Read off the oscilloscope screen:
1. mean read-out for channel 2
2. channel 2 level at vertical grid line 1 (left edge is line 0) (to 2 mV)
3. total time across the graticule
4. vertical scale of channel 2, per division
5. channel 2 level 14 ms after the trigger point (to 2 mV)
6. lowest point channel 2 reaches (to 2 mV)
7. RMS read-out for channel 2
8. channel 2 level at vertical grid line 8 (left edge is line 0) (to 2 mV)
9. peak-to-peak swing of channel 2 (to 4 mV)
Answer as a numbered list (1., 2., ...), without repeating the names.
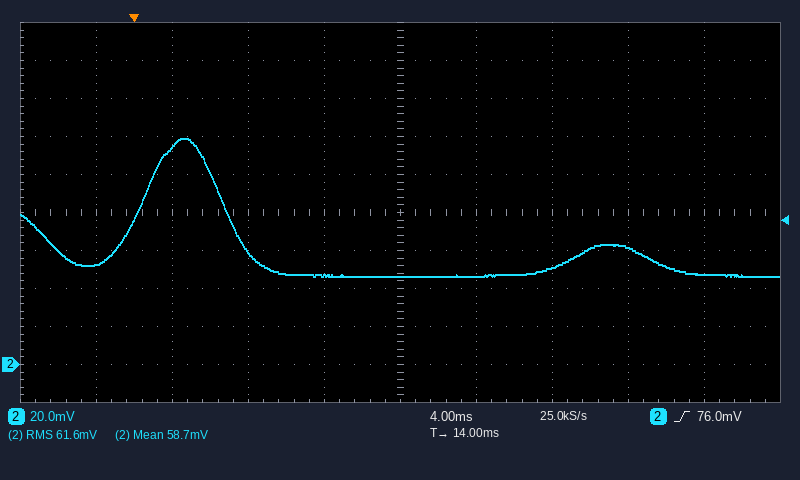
1. 58.7 mV
2. 52 mV
3. 40 ms
4. 20 mV
5. 46 mV
6. 46 mV
7. 61.6 mV
8. 62 mV
9. 72 mV
